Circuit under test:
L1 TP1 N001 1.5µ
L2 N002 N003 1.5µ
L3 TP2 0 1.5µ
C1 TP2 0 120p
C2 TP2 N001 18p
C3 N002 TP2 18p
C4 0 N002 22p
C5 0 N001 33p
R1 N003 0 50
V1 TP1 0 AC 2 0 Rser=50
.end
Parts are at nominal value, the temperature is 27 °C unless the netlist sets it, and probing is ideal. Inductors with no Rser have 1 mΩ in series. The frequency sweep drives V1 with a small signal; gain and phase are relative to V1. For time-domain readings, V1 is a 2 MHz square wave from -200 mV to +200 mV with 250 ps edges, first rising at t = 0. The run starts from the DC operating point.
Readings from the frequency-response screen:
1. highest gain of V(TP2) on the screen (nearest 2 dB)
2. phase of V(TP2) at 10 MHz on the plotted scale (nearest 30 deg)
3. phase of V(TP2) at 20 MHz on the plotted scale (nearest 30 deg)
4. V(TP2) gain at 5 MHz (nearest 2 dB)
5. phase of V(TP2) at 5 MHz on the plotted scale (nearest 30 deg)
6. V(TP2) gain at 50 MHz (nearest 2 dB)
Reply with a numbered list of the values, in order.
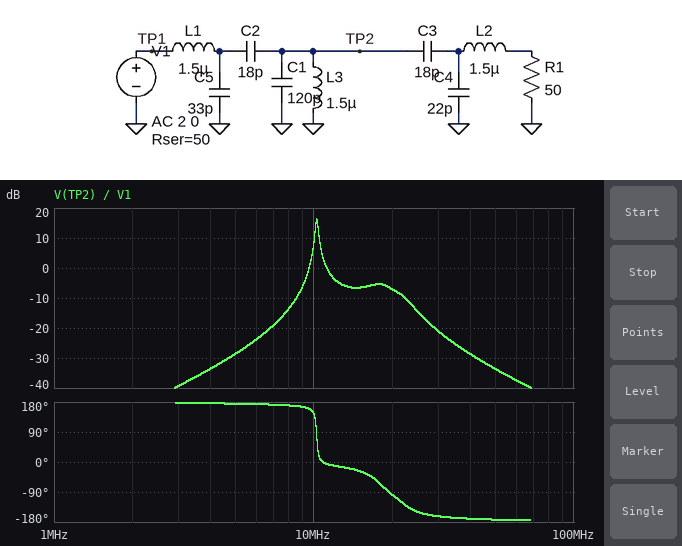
1. 16 dB
2. 150 deg
3. -90 deg
4. -28 dB
5. 180 deg
6. -34 dB
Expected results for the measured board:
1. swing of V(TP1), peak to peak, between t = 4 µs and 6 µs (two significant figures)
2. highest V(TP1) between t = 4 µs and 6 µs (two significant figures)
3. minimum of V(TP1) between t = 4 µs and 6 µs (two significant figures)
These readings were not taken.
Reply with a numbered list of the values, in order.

1. 520 mV
2. 260 mV
3. -260 mV
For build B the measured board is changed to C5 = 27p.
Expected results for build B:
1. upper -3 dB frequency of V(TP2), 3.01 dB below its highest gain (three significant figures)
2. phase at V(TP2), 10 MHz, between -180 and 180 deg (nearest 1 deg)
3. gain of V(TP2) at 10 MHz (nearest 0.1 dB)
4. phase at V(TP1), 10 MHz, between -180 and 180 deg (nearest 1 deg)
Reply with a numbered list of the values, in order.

1. 10.4 MHz
2. 146 deg
3. 8.5 dB
4. -22 deg
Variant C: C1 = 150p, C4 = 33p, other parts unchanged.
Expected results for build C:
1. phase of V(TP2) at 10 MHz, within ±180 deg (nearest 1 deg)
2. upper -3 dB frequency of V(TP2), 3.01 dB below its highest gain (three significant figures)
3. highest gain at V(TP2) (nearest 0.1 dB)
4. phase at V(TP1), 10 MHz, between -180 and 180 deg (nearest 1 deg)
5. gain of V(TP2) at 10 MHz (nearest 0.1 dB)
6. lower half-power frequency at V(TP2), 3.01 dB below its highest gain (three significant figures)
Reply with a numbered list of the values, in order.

1. -3 deg
2. 9.51 MHz
3. 16.9 dB
4. -8 deg
5. 1.1 dB
6. 9.35 MHz
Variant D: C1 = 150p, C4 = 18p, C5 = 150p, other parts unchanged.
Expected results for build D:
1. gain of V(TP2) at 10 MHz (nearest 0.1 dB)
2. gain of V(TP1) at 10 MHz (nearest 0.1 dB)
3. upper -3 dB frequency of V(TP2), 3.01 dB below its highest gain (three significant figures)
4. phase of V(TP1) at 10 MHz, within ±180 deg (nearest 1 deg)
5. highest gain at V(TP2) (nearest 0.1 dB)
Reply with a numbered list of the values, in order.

1. 5.4 dB
2. -13.6 dB
3. 9.64 MHz
4. -73 deg
5. 16.7 dB
